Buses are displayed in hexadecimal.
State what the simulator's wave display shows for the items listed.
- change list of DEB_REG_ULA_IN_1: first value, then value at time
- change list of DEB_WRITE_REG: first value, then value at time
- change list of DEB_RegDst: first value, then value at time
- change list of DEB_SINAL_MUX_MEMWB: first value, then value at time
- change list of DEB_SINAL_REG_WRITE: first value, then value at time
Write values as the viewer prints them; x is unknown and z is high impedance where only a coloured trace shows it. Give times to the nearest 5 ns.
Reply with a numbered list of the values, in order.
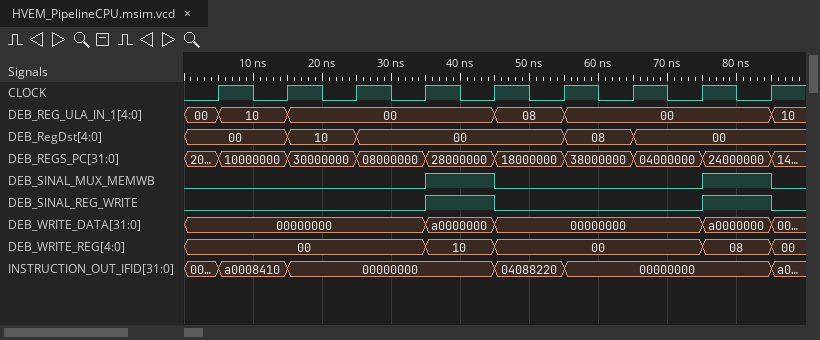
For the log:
1. 00, 10 at 5 ns, 00 at 15 ns, 08 at 45 ns, 00 at 55 ns, 10 at 85 ns
2. 00, 10 at 35 ns, 00 at 45 ns, 08 at 75 ns, 00 at 85 ns
3. 00, 10 at 15 ns, 00 at 25 ns, 08 at 55 ns, 00 at 65 ns
4. 0, 1 at 35 ns, 0 at 45 ns, 1 at 75 ns, 0 at 85 ns
5. 0, 1 at 35 ns, 0 at 45 ns, 1 at 75 ns, 0 at 85 ns
